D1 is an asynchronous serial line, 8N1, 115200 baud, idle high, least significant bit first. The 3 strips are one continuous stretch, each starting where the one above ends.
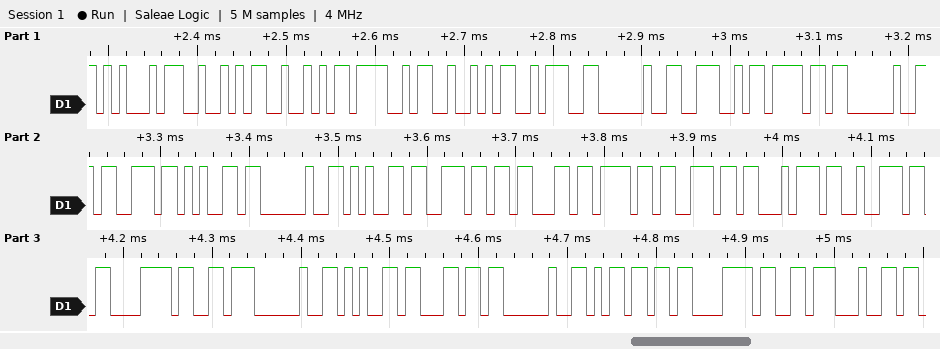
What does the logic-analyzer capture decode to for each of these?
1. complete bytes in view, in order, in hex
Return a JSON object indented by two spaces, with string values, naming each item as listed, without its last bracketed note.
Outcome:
{
  "complete bytes in view, in order, in hex": "45 52 52 4F 52 3A 20 4E 6F 20 73 65 20 65 6E 63 6F 6E 74 72 C3 B3 20 65 6C 20 6D C3 B3 64"
}
